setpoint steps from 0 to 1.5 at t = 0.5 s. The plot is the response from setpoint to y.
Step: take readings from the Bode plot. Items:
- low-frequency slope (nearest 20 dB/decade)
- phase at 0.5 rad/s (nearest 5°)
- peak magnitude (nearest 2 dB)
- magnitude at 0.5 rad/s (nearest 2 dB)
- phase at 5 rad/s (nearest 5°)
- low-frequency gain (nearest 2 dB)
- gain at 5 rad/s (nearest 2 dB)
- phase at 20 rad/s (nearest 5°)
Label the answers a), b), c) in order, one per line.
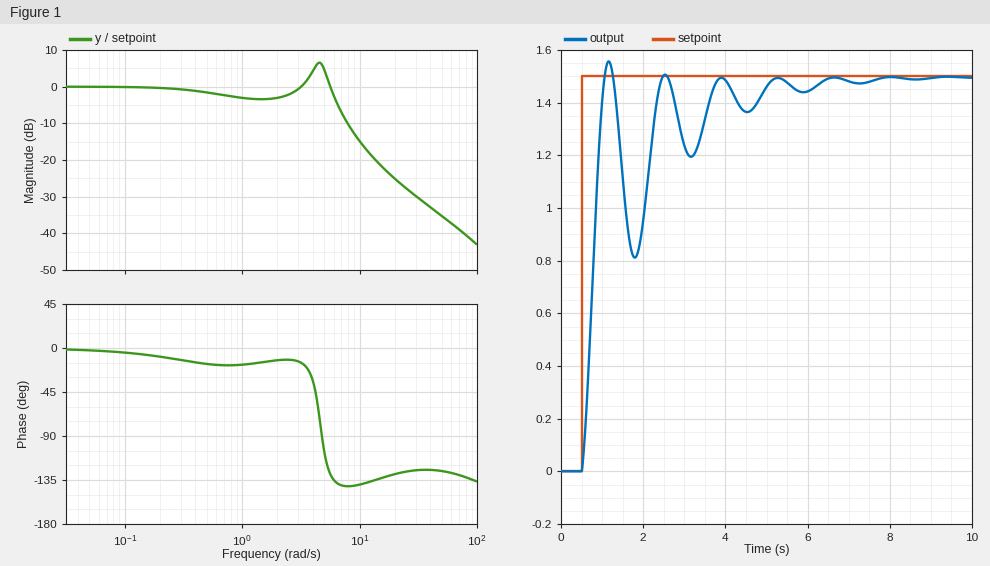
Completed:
a) 0 dB/decade
b) -15°
c) 6 dB
d) -2 dB
e) -105°
f) 0 dB
g) 4 dB
h) -130°
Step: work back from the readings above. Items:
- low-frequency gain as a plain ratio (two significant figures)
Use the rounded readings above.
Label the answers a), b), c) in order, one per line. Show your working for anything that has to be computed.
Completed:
a) 10^(0 / 20) = 1.0
